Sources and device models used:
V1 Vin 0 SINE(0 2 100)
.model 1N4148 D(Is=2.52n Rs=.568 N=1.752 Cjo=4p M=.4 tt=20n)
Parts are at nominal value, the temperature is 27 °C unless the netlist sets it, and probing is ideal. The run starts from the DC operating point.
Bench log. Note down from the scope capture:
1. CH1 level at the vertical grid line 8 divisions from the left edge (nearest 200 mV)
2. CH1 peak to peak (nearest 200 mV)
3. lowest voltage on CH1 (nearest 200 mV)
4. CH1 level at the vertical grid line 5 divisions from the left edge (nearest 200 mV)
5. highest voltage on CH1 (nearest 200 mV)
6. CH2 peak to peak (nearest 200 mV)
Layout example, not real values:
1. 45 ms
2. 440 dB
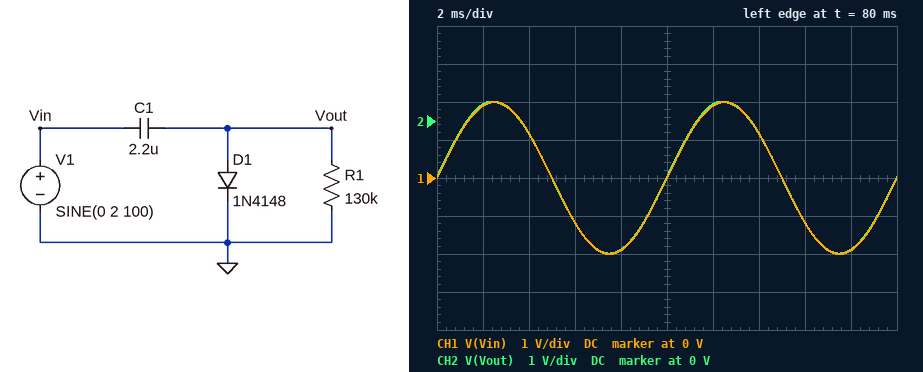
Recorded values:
1. -1.2 V
2. 4.0 V
3. -2.0 V
4. 0 V
5. 2.0 V
6. 4.0 V
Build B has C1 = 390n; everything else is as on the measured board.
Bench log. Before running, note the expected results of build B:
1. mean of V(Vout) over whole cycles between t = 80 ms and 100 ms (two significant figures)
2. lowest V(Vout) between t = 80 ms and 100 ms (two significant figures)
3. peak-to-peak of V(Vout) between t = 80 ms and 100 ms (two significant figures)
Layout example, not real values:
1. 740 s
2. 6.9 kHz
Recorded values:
1. -1.4 V
2. -3.4 V
3. 3.9 V
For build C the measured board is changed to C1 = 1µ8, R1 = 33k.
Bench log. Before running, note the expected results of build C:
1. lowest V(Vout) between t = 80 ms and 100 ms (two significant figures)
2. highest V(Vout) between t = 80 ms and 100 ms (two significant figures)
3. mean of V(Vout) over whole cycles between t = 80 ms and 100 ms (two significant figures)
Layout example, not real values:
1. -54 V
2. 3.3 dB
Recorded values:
1. -3.4 V
2. 560 mV
3. -1.4 V
